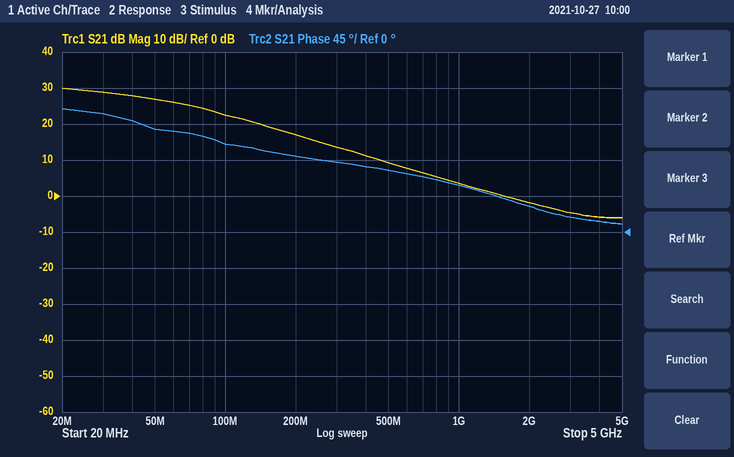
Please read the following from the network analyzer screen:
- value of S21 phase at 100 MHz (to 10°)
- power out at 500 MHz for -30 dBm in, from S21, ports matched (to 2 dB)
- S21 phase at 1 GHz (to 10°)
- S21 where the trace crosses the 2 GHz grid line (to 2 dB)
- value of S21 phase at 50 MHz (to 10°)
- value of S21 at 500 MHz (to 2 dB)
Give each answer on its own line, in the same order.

110°
-20 dBm
60°
-2 dB
130°
10 dB
